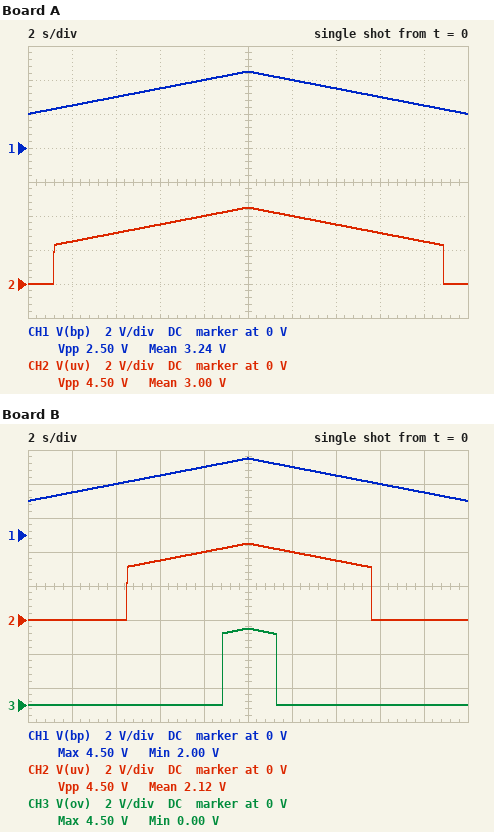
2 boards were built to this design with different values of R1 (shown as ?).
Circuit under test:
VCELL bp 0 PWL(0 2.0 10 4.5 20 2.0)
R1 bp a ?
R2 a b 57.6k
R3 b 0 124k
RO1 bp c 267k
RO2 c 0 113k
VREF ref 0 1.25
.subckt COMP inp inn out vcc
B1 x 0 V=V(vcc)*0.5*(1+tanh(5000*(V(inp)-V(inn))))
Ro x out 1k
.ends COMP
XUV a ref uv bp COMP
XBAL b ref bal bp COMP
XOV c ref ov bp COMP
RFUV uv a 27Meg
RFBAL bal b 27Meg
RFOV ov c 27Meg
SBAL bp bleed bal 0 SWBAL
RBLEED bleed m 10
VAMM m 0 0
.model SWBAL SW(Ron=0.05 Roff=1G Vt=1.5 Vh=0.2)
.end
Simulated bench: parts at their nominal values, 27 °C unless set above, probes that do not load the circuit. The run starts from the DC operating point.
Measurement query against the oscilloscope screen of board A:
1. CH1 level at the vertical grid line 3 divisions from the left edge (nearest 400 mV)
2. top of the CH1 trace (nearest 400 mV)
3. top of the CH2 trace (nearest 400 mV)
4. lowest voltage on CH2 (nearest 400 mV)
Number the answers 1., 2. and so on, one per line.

1. 3.6 V
2. 4.4 V
3. 4.4 V
4. 0 V
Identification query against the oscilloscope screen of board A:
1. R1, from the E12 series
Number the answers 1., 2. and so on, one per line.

1. 150 kΩ
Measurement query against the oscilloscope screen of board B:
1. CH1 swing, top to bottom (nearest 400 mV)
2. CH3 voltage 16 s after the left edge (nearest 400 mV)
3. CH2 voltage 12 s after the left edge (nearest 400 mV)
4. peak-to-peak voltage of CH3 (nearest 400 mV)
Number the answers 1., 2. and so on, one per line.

1. 2.4 V
2. 0 V
3. 4.0 V
4. 4.4 V
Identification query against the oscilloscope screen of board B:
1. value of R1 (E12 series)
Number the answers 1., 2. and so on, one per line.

1. 270 kΩ
